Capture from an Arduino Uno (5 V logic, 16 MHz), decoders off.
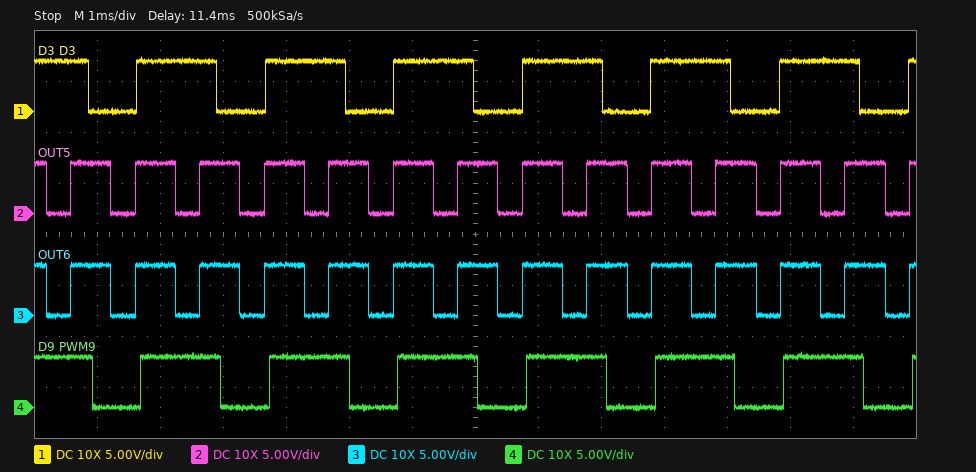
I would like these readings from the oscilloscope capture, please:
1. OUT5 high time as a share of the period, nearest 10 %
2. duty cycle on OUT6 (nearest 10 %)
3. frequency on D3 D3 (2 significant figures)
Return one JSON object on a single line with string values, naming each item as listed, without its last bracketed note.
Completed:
{"OUT5 high time as a share of the period, nearest 10 %": "60 %", "duty cycle on OUT6": "60 %", "frequency on D3 D3": "490 Hz"}
